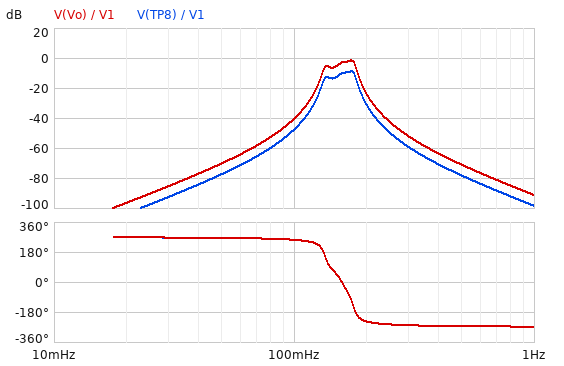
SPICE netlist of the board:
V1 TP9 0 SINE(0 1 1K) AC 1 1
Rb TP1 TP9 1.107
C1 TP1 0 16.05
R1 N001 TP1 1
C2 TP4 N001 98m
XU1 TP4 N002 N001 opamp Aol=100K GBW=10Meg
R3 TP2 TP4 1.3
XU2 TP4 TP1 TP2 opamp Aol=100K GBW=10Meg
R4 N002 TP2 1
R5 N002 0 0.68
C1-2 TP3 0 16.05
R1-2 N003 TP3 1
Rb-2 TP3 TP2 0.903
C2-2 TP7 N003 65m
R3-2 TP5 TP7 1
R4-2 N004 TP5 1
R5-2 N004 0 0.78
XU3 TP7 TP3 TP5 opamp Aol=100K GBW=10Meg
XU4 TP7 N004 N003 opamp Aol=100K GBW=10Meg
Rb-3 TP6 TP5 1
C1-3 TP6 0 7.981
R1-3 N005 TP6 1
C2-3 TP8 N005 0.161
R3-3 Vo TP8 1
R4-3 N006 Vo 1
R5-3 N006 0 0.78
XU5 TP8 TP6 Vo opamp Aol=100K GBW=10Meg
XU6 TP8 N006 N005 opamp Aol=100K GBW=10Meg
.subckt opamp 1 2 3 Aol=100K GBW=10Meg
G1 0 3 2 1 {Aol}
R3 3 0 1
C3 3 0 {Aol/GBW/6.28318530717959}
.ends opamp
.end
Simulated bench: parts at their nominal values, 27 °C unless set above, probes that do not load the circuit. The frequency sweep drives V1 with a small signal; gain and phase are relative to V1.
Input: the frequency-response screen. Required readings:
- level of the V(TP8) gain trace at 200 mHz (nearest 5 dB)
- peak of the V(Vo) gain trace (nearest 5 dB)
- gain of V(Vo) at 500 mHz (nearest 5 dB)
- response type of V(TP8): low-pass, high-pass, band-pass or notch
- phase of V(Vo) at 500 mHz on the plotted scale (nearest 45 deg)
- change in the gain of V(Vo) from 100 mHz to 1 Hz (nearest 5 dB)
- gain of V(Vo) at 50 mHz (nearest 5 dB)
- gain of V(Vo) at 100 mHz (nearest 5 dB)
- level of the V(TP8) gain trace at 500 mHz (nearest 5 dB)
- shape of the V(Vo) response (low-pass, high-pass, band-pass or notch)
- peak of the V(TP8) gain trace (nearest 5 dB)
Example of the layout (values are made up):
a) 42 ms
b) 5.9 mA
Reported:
a) -30 dB
b) 0 dB
c) -70 dB
d) band-pass
e) -270 deg
f) -50 dB
g) -70 dB
h) -40 dB
i) -80 dB
j) band-pass
k) -10 dB
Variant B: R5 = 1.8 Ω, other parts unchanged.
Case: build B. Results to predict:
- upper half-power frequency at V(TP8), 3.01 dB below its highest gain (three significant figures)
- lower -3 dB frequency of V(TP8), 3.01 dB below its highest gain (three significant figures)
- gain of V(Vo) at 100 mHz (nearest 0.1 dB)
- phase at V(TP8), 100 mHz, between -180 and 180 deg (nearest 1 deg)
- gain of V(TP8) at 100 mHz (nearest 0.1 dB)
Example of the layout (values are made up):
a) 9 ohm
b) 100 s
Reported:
a) 180 mHz
b) 162 mHz
c) -36.5 dB
d) 96 deg
e) -43.6 dB
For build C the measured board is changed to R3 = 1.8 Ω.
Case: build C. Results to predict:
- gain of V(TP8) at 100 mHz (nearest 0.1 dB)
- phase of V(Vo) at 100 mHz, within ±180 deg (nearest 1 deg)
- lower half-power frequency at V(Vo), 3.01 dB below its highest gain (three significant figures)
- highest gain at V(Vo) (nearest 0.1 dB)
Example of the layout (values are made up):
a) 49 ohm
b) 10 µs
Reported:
a) -39.7 dB
b) -116 deg
c) 159 mHz
d) -4.4 dB
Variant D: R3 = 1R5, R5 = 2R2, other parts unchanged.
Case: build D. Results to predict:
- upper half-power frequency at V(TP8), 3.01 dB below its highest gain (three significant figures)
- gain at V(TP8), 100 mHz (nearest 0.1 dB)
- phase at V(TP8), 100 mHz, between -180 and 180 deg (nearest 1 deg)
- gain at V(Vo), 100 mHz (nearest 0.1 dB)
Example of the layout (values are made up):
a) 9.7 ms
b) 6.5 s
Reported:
a) 180 mHz
b) -48.3 dB
c) 89 deg
d) -41.1 dB
